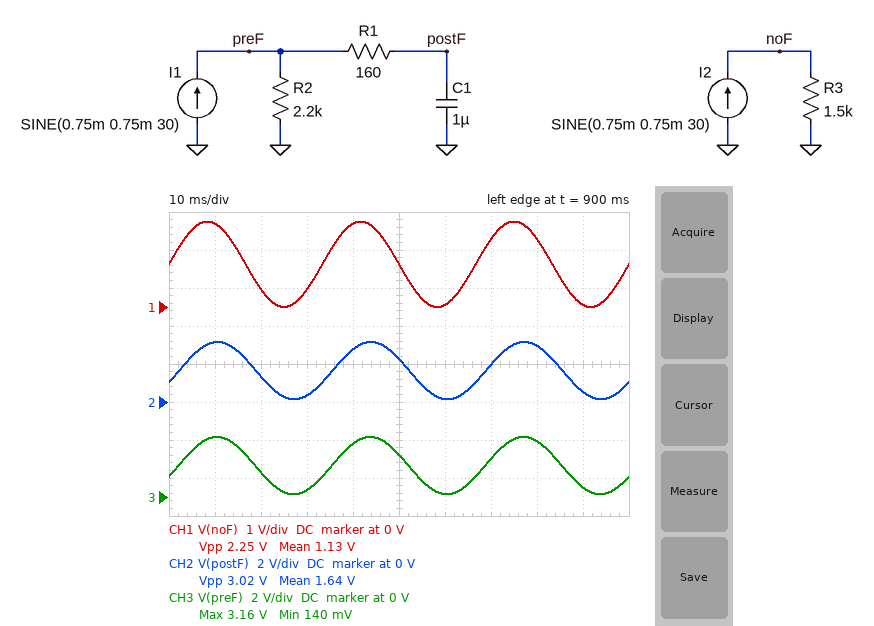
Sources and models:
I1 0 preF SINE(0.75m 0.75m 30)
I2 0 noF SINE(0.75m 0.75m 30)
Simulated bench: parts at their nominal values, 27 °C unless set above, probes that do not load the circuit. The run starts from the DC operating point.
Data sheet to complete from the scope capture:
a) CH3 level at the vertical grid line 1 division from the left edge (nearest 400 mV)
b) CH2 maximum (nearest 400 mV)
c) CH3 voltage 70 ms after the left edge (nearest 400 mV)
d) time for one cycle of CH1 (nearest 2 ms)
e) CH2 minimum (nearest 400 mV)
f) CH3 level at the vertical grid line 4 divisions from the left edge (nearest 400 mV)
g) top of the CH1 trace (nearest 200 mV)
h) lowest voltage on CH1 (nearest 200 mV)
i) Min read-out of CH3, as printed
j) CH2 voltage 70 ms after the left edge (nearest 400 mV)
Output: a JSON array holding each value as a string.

["3.2 V", "3.2 V", "2.0 V", "34 ms", "0 V", "2.8 V", "2.2 V", "0 V", "140 mV", "2.0 V"]
